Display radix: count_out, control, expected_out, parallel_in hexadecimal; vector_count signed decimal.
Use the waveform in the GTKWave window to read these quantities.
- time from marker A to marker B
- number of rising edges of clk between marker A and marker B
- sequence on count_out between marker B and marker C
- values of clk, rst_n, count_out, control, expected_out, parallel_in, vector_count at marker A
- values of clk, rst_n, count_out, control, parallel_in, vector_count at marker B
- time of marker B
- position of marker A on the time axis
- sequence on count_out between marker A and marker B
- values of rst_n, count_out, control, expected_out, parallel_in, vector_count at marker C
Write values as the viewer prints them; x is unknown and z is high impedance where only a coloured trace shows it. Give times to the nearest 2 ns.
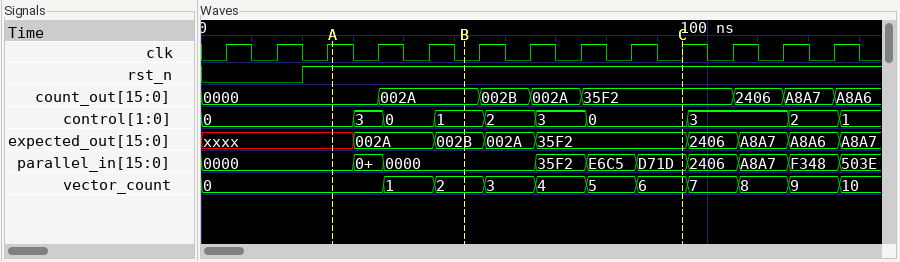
26 ns
2
002A, 002B, 002A, 35F2
clk=1, rst_n=1, count_out=0000, control=0, expected_out=xxxx, parallel_in=0000, vector_count=0
clk=0, rst_n=1, count_out=002A, control=1, parallel_in=0000, vector_count=2
52 ns
26 ns
0000, 002A
rst_n=1, count_out=35F2, control=0, expected_out=35F2, parallel_in=D71D, vector_count=6
